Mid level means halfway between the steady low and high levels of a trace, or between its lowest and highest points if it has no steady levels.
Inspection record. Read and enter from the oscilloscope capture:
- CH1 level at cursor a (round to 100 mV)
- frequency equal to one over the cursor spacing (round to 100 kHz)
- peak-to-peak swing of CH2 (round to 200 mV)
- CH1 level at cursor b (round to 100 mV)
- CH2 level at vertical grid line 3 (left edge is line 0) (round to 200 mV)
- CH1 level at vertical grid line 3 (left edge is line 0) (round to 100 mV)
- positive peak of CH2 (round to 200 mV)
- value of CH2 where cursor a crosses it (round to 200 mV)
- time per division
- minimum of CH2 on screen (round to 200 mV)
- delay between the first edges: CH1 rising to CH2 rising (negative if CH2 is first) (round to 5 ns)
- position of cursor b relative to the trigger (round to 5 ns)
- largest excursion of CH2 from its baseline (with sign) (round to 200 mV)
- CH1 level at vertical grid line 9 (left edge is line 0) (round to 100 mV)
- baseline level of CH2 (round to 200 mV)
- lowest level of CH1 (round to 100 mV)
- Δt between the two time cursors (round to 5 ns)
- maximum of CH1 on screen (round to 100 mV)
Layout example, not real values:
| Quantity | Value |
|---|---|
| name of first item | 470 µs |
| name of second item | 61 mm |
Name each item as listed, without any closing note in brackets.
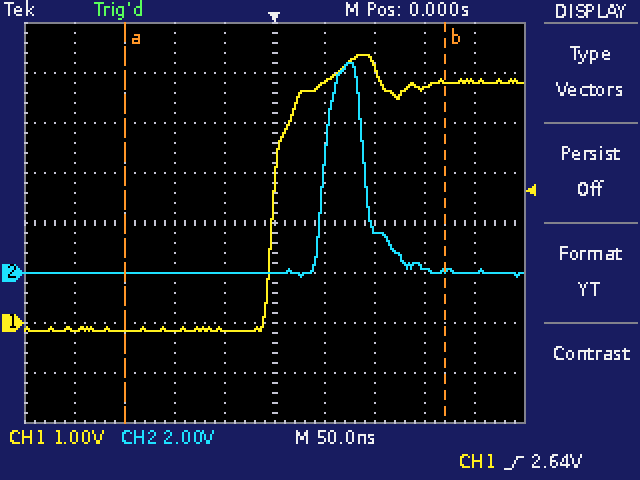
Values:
| Quantity | Value |
|---|---|
| CH1 level at cursor a | -200 mV |
| frequency equal to one over the cursor spacing | 3.1 MHz |
| peak-to-peak swing of CH2 | 8.6 V |
| CH1 level at cursor b | 4.8 V |
| CH2 level at vertical grid line 3 (left edge is line 0) | 0.0 V |
| CH1 level at vertical grid line 3 (left edge is line 0) | -200 mV |
| positive peak of CH2 | 8.4 V |
| value of CH2 where cursor a crosses it | 0.0 V |
| time per division | 50 ns |
| minimum of CH2 on screen | -200 mV |
| delay between the first edges: CH1 rising to CH2 rising (negative if CH2 is first) | +50 ns |
| position of cursor b relative to the trigger | +170 ns |
| largest excursion of CH2 from its baseline (with sign) | +8.4 V |
| CH1 level at vertical grid line 9 (left edge is line 0) | 4.8 V |
| baseline level of CH2 | 0.0 V |
| lowest level of CH1 | -200 mV |
| Δt between the two time cursors | 320 ns |
| maximum of CH1 on screen | 5.4 V |
